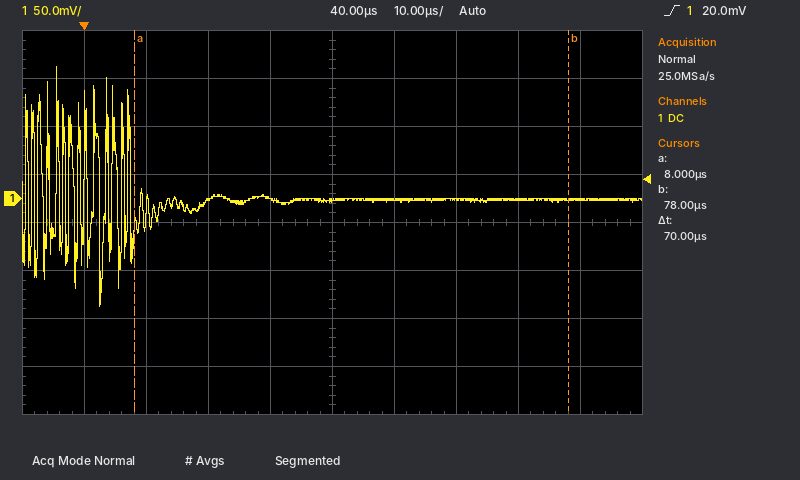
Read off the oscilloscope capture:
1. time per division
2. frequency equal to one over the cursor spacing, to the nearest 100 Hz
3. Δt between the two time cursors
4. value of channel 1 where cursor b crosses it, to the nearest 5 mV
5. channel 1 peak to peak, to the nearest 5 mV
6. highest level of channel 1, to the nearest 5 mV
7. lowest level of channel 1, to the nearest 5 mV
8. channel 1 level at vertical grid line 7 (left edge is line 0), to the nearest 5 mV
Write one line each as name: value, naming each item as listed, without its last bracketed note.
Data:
time per division: 10 µs
frequency equal to one over the cursor spacing, to the nearest 100 Hz: 14.3 kHz
Δt between the two time cursors: 70 µs
value of channel 1 where cursor b crosses it, to the nearest 5 mV: 0 mV
channel 1 peak to peak, to the nearest 5 mV: 250 mV
highest level of channel 1, to the nearest 5 mV: 140 mV
lowest level of channel 1, to the nearest 5 mV: -110 mV
channel 1 level at vertical grid line 7 (left edge is line 0), to the nearest 5 mV: 0 mV
